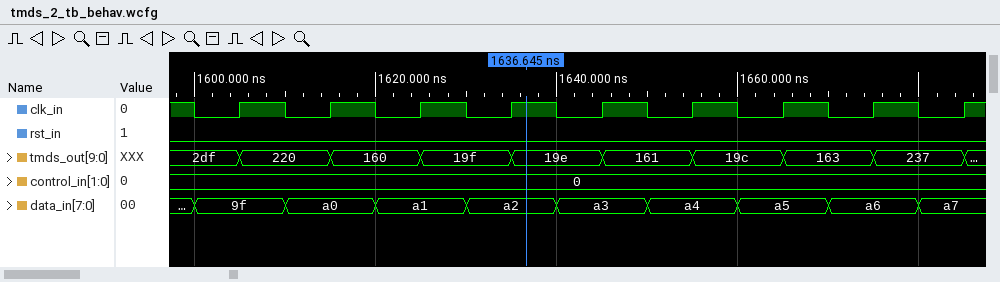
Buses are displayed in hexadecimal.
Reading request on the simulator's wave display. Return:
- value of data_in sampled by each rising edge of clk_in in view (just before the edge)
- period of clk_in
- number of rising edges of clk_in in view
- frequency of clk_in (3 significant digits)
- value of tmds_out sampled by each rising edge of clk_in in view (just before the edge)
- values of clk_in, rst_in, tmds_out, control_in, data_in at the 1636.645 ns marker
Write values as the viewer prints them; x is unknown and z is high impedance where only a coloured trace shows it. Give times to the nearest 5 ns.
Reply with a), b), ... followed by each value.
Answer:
a) 9f, a0, a1, a2, a3, a4, a5, a6, a7
b) 10 ns
c) 9
d) 100 MHz
e) 2df, 220, 160, 19f, 19e, 161, 19c, 163, 237
f) clk_in=1, rst_in=0, tmds_out=19e, control_in=0, data_in=a2
